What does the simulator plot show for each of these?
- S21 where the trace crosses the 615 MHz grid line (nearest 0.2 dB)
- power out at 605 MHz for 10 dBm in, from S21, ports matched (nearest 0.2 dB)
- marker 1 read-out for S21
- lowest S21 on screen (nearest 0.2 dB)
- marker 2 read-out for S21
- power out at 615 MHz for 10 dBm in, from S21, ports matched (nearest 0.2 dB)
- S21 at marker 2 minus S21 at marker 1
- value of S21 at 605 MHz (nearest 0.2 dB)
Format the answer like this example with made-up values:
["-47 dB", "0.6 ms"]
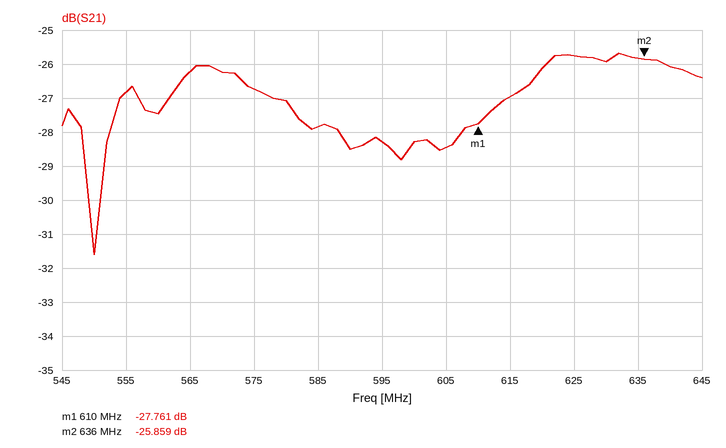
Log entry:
["-27.0 dB", "-18.4 dBm", "-27.761 dB", "-31.6 dB", "-25.859 dB", "-17.0 dBm", "1.902 dB", "-28.4 dB"]
